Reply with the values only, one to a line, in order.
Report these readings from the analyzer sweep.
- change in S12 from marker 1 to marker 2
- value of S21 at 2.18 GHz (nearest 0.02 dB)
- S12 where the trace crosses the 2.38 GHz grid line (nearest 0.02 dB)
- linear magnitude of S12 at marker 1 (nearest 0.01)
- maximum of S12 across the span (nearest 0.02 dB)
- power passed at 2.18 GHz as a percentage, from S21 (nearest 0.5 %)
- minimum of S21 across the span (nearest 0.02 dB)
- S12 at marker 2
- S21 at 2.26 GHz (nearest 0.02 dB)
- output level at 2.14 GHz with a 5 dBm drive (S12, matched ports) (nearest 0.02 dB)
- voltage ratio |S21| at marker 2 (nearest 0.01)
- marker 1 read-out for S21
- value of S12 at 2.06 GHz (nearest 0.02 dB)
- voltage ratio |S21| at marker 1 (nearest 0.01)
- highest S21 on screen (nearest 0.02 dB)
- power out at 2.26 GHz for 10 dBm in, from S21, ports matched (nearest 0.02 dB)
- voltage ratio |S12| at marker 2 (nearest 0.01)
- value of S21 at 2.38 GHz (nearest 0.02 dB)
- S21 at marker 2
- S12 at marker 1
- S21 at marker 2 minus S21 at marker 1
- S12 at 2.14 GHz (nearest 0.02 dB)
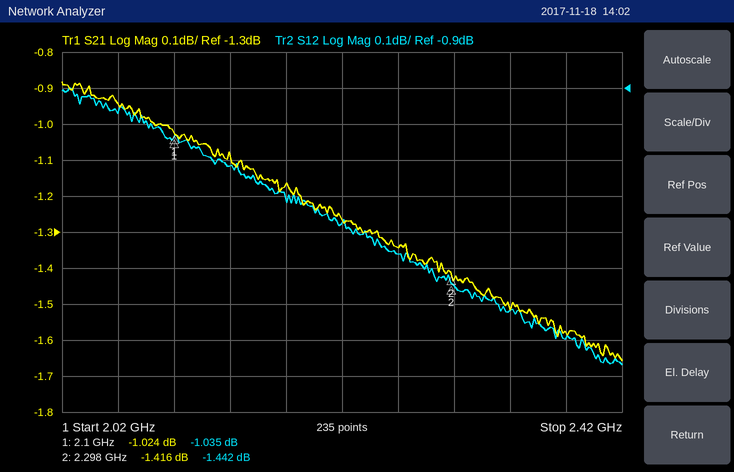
-0.407 dB
-1.16 dB
-1.60 dB
0.89
-0.90 dB
76.5 %
-1.66 dB
-1.442 dB
-1.34 dB
3.88 dBm
0.85
-1.024 dB
-0.96 dB
0.89
-0.88 dB
8.66 dBm
0.85
-1.58 dB
-1.416 dB
-1.035 dB
-0.392 dB
-1.12 dB
